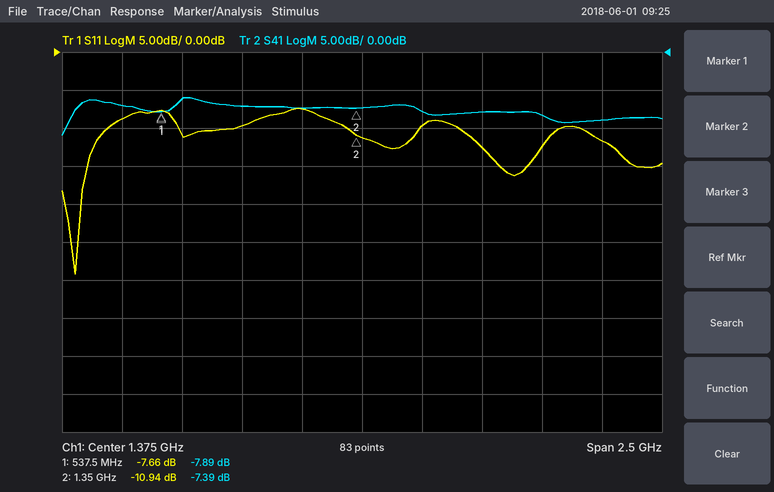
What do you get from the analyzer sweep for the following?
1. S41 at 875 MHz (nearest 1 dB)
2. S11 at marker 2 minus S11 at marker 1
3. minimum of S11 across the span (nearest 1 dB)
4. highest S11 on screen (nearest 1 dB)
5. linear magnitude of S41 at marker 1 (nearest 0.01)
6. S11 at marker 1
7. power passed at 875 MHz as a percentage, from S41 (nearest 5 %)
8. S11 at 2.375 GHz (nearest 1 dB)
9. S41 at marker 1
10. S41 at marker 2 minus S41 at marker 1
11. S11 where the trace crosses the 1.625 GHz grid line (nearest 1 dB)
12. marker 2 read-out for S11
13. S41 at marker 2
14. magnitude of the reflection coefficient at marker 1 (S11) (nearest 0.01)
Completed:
-7 dB
-3.28 dB
-29 dB
-7 dB
0.40
-7.66 dB
20 %
-12 dB
-7.89 dB
0.50 dB
-10 dB
-10.94 dB
-7.39 dB
0.41
